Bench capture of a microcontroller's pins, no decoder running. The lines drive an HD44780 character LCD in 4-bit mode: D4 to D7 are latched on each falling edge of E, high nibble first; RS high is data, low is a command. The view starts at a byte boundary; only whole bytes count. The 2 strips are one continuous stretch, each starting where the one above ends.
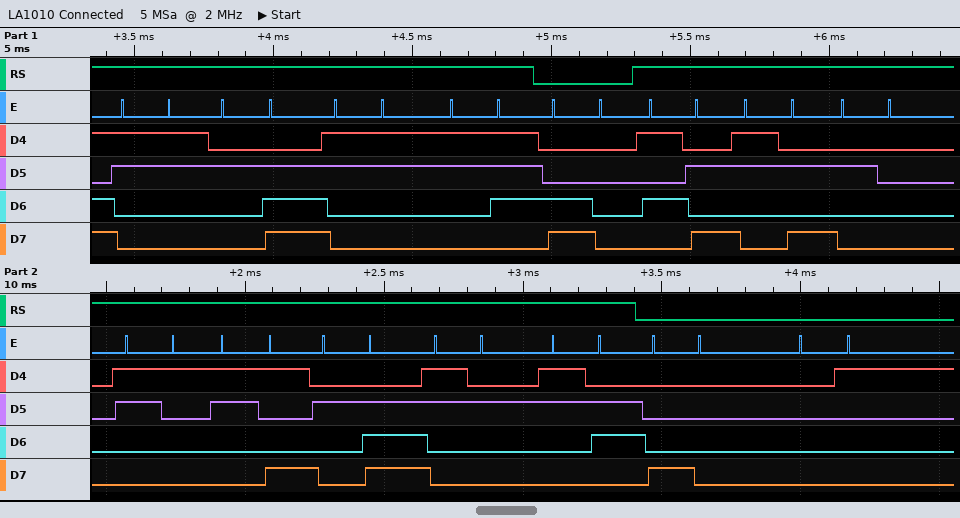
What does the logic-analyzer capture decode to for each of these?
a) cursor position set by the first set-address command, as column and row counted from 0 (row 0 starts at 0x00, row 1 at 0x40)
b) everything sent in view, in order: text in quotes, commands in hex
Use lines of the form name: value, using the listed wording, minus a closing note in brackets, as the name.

cursor position set by the first set-address command, as column and row counted from 0: column 0, row 1
everything sent in view, in order: text in quotes, commands in hex: "3.37" 0xC0 "Z: 19.26" 0x80 0x01
